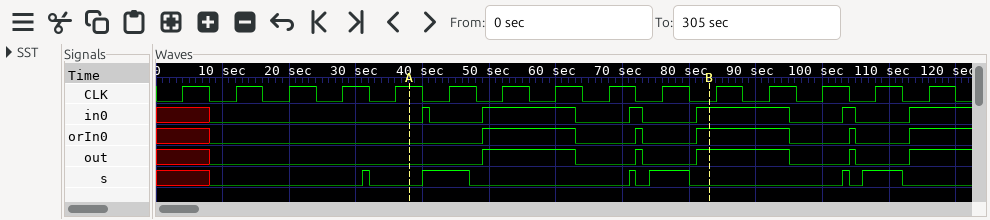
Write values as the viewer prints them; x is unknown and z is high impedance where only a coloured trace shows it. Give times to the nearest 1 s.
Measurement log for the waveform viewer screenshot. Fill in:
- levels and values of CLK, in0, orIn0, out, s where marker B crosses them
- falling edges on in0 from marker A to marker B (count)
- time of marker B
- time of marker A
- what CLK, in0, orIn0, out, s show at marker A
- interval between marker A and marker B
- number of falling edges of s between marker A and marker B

CLK=0, in0=1, orIn0=1, out=1, s=0
3
83 s
38 s
CLK=1, in0=0, orIn0=0, out=0, s=0
45 s
3
